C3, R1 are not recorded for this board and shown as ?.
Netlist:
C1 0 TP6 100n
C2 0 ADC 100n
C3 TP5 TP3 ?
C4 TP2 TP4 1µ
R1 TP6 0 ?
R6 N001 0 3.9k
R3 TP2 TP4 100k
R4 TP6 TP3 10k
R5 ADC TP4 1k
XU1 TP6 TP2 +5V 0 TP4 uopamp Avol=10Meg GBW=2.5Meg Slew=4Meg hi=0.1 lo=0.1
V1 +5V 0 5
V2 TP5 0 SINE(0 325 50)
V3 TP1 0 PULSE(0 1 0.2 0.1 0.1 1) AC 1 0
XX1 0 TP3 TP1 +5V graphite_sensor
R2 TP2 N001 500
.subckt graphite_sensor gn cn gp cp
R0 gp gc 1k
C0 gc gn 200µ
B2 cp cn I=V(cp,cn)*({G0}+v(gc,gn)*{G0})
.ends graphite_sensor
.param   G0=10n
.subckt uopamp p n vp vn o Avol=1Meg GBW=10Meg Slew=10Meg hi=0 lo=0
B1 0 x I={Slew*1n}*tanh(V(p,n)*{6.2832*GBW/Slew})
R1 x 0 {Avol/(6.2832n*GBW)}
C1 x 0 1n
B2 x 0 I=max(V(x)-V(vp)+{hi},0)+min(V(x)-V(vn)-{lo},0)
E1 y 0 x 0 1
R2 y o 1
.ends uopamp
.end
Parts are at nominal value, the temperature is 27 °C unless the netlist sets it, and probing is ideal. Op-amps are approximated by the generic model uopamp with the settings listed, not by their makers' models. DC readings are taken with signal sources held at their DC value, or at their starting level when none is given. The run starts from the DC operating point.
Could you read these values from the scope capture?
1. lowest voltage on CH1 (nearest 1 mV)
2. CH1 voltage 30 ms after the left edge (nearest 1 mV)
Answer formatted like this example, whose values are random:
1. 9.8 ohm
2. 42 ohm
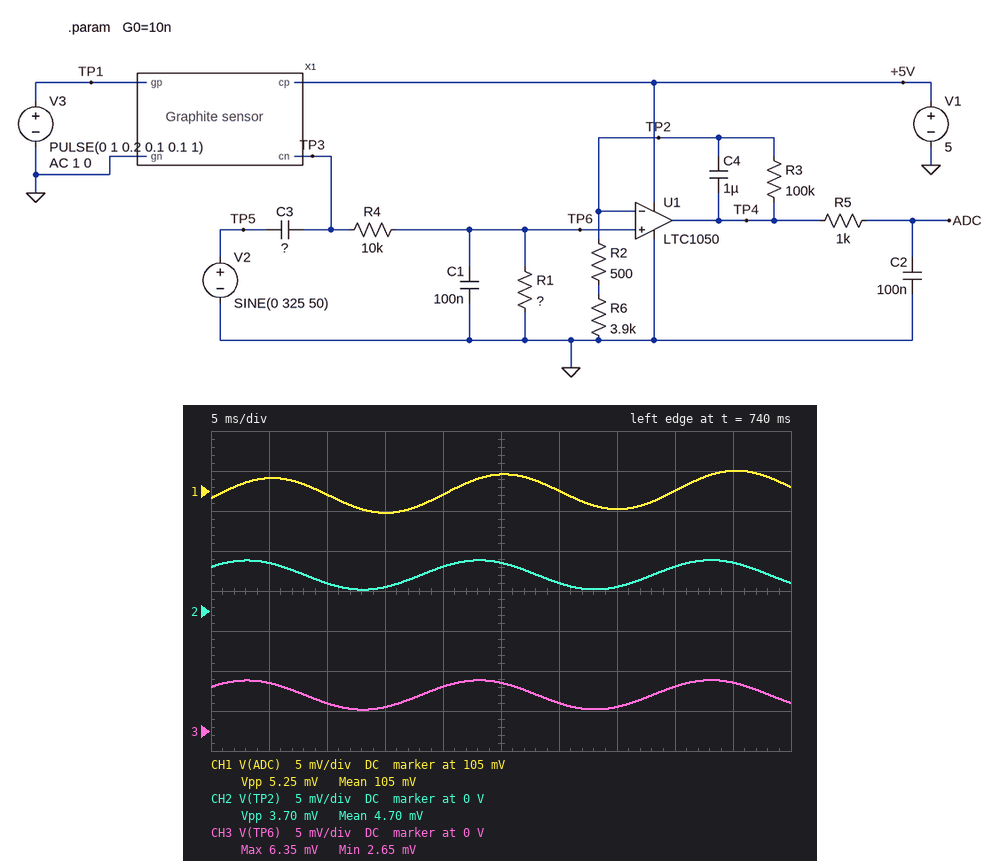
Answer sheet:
1. 102 mV
2. 105 mV
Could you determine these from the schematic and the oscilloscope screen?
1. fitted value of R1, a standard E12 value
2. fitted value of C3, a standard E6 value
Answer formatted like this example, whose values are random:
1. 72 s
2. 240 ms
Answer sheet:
1. 47 kΩ
2. 680 fF
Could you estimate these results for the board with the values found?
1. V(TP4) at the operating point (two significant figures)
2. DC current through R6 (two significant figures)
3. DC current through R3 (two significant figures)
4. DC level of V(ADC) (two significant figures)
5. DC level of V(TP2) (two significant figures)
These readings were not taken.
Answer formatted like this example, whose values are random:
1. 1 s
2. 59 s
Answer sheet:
1. 100 mV
2. 960 nA
3. 960 nA
4. 100 mV
5. 4.2 mV
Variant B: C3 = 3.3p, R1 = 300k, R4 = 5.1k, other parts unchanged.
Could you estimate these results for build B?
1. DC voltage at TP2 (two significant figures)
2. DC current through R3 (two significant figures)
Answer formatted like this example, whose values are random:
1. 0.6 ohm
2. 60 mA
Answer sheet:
1. 15 mV
2. 3.4 µA
